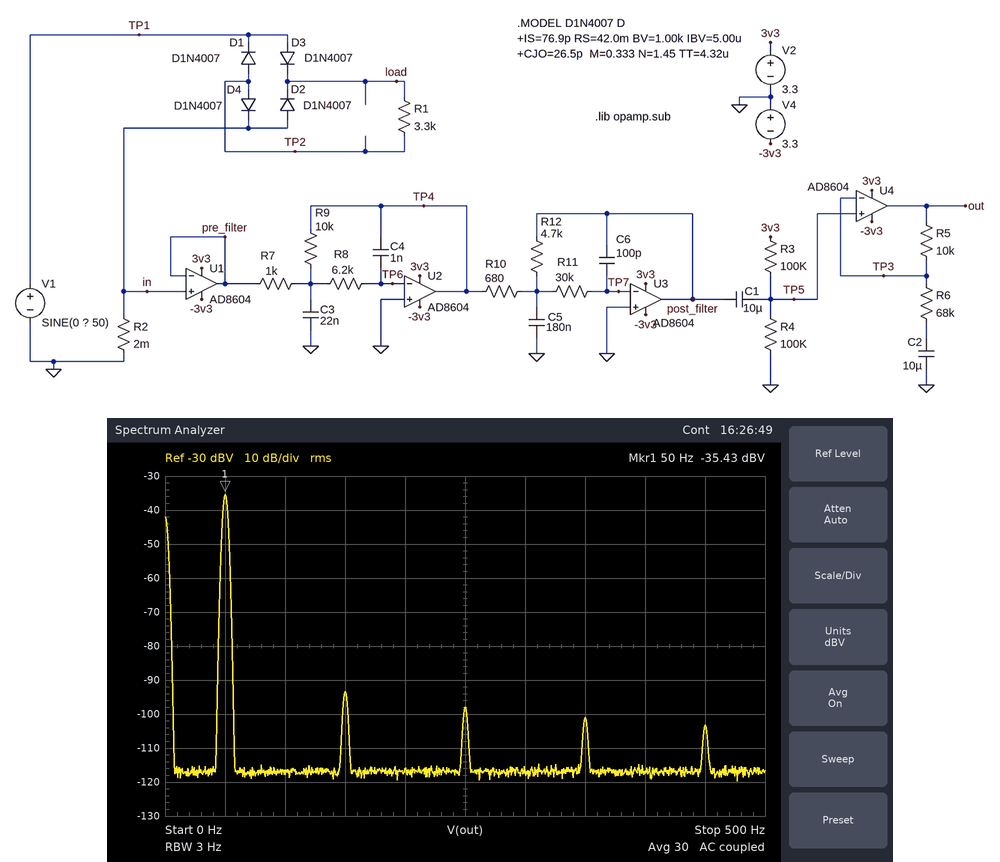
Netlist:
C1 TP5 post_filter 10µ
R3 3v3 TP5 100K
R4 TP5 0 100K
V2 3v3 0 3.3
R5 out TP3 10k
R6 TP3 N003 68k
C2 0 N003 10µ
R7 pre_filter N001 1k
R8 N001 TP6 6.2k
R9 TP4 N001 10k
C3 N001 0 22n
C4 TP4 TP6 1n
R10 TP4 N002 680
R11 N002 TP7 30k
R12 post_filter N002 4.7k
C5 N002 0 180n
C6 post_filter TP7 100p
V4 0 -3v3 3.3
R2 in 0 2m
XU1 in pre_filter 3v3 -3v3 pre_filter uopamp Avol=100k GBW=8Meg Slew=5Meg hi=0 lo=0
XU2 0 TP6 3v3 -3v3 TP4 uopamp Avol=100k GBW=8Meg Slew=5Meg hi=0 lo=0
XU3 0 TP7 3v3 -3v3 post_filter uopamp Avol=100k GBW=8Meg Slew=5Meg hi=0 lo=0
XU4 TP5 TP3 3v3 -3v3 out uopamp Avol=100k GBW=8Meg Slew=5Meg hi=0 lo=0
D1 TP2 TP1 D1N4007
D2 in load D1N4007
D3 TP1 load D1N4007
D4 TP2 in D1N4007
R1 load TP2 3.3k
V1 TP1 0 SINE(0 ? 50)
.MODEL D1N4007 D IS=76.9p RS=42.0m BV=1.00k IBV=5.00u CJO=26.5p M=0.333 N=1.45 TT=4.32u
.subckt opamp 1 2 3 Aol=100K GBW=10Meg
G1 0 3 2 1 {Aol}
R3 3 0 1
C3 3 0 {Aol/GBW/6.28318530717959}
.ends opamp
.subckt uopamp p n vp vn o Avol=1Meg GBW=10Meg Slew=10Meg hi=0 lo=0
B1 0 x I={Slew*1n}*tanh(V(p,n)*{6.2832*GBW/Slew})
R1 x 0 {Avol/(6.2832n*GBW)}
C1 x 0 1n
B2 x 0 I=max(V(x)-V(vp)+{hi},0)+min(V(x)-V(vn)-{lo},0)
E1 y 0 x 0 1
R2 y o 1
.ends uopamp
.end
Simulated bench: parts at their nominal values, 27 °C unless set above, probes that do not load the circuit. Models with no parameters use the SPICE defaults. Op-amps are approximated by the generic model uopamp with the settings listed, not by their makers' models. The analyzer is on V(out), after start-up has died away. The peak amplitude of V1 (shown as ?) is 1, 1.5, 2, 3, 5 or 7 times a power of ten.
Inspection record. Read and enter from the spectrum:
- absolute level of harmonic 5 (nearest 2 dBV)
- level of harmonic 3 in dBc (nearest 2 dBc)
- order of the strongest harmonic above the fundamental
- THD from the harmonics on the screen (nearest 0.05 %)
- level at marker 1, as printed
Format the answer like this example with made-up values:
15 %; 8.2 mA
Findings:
-98 dBV; -58 dBc; 3; 0.15 %; -35.43 dBV
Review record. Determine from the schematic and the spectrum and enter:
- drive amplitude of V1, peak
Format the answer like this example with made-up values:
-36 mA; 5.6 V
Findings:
500 V
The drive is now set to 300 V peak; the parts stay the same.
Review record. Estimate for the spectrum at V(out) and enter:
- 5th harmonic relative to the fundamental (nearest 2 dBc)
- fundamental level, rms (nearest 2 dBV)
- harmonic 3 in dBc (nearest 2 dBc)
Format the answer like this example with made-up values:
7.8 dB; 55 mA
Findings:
-58 dBc; -40 dBV; -54 dBc
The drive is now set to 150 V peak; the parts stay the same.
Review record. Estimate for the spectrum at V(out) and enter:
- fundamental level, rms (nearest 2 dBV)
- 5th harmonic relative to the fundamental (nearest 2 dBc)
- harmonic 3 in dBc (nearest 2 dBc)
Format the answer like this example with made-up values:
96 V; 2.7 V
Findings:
-46 dBV; -52 dBc; -48 dBc
